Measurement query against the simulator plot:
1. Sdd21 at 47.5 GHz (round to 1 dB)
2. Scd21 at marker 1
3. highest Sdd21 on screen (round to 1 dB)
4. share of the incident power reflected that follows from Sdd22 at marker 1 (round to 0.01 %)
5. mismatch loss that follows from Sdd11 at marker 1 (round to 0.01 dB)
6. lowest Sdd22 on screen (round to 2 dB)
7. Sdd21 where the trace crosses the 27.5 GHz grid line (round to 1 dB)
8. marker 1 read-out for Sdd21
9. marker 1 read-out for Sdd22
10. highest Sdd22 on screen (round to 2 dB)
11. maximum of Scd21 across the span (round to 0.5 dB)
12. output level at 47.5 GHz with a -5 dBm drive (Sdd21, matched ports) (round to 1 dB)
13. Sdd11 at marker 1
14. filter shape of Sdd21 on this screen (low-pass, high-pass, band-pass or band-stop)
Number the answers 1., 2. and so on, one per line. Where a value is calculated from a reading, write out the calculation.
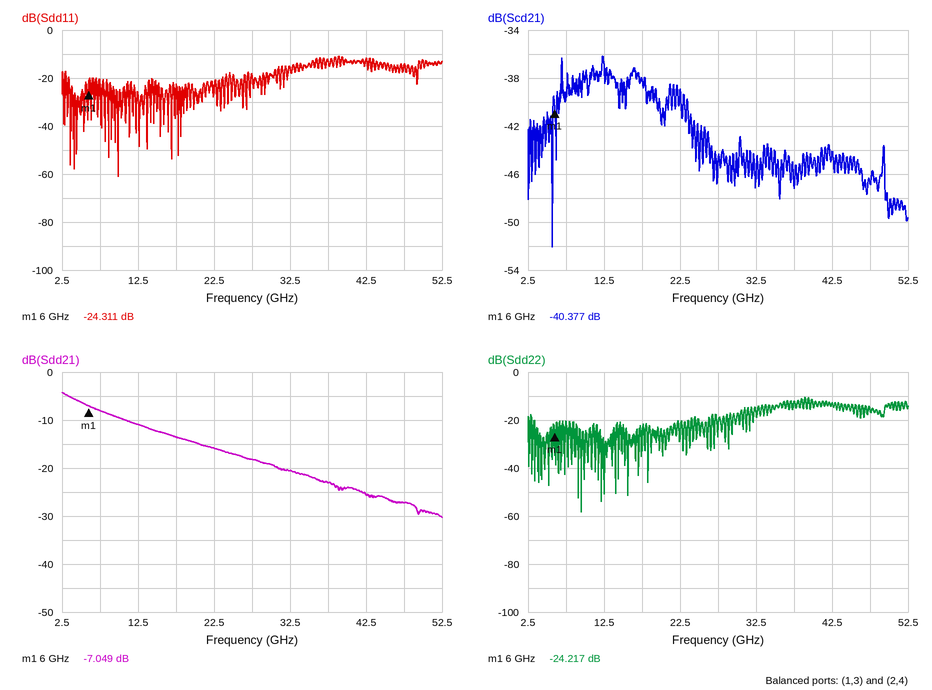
1. -27 dB
2. -40.377 dB
3. -4 dB
4. 10^(-24.217/10) ≈ 0.38 %
5. −10 log10(1 − 10^(-24.311/10)) ≈ 0.02 dB
6. -58 dB
7. -18 dB
8. -7.049 dB
9. -24.217 dB
10. -10 dB
11. -36.0 dB
12. -5 dBm + (-27 dB) = -32 dBm
13. -24.311 dB
14. low-pass
